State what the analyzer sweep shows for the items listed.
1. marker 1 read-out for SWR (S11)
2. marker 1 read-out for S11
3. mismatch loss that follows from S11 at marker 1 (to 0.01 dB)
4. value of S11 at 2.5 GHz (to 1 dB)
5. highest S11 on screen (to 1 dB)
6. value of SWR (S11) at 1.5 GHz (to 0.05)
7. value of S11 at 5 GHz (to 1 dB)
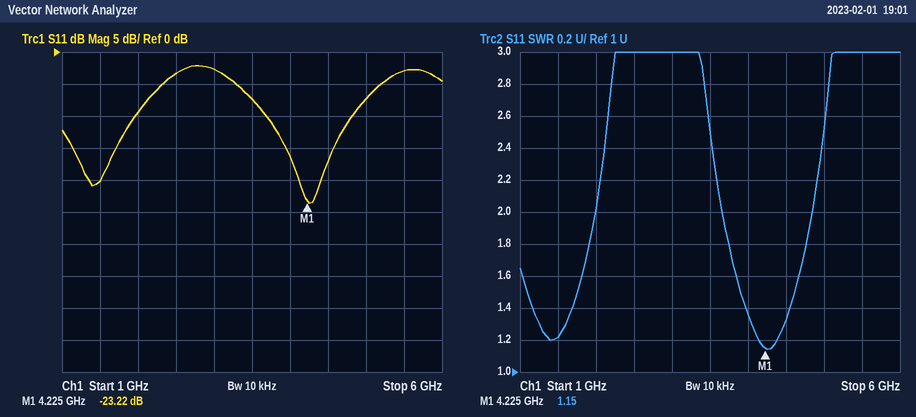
1.15
-23.22 dB
0.02 dB
-3 dB
-2 dB
1.20
-7 dB
